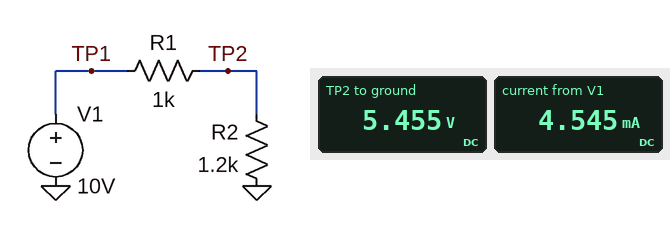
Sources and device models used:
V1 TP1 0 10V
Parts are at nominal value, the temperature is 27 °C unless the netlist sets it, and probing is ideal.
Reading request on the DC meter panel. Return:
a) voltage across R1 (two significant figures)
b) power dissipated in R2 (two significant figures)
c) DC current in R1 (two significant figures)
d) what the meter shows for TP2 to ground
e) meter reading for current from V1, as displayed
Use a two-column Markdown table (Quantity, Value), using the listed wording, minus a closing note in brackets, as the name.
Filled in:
| Quantity | Value |
|---|---|
| voltage across R1 | 4.5 V |
| power dissipated in R2 | 25 mW |
| DC current in R1 | 4.5 mA |
| what the meter shows for TP2 to ground | 5.455 V |
| meter reading for current from V1, as displayed | 4.545 mA |
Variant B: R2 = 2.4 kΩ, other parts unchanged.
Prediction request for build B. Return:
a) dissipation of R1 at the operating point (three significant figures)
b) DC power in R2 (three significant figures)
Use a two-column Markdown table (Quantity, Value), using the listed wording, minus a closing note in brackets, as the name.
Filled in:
| Quantity | Value |
|---|---|
| dissipation of R1 at the operating point | 8.65 mW |
| DC power in R2 | 20.8 mW |
